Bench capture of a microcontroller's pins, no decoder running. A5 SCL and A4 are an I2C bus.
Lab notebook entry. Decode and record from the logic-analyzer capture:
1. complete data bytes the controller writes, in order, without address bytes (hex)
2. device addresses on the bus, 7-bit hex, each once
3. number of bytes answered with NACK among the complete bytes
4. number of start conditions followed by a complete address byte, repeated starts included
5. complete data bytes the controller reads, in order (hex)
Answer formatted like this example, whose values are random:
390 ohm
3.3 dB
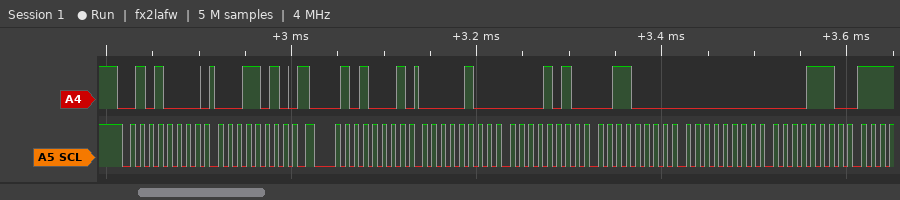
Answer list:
1A
0x28
0
2
04 0A 30 00 0E
